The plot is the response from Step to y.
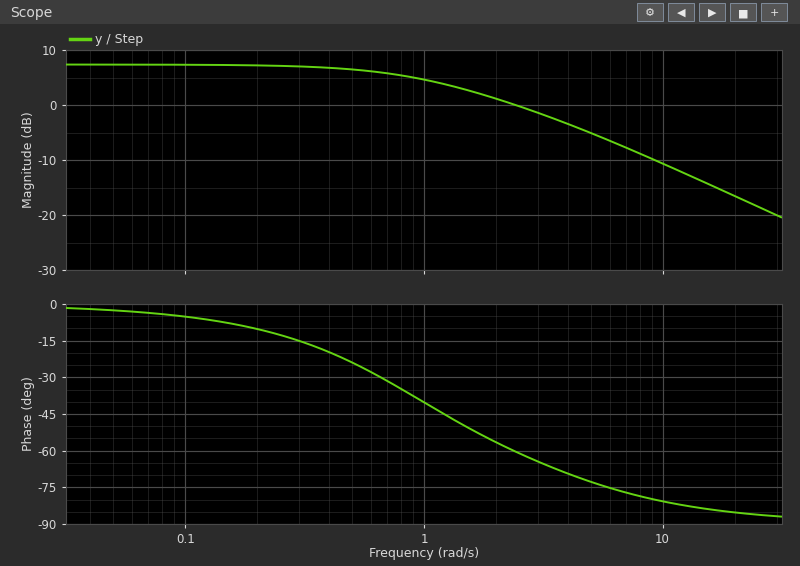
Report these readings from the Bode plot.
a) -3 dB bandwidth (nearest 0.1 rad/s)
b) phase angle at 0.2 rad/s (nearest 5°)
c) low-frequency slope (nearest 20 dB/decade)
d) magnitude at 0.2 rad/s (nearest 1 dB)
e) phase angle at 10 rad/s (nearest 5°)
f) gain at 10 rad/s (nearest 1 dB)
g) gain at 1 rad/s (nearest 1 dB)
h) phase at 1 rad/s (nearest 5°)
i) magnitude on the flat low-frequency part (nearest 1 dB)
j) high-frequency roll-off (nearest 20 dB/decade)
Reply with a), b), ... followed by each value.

a) 1.1 rad/s
b) -10°
c) 0 dB/decade
d) 7 dB
e) -80°
f) -11 dB
g) 5 dB
h) -40°
i) 7 dB
j) -20 dB/decade
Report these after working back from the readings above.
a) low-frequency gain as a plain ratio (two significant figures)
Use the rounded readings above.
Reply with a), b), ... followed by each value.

a) 2.2
